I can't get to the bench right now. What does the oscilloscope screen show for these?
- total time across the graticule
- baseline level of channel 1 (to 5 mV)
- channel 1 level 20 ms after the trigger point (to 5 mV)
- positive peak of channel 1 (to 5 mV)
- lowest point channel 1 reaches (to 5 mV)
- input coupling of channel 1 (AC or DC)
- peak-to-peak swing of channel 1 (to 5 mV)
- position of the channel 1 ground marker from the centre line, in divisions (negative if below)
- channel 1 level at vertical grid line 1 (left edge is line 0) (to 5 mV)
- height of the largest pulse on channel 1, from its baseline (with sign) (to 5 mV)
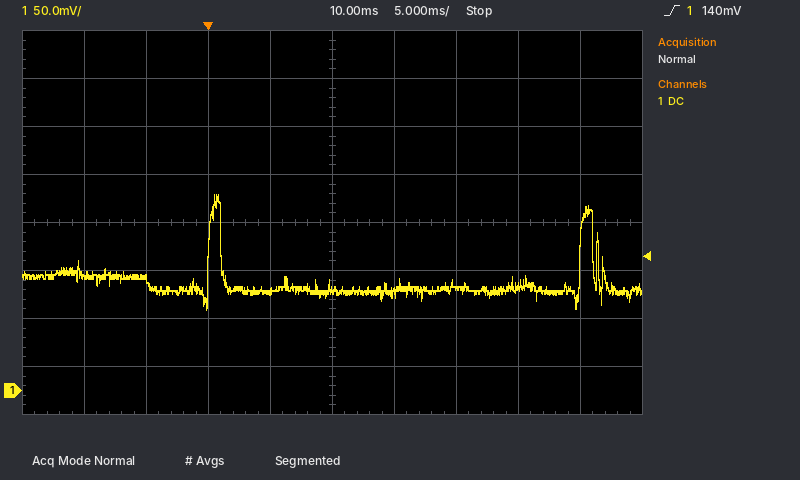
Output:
50 ms
105 mV
105 mV
205 mV
85 mV
DC
120 mV
-3.5 div
120 mV
+100 mV
